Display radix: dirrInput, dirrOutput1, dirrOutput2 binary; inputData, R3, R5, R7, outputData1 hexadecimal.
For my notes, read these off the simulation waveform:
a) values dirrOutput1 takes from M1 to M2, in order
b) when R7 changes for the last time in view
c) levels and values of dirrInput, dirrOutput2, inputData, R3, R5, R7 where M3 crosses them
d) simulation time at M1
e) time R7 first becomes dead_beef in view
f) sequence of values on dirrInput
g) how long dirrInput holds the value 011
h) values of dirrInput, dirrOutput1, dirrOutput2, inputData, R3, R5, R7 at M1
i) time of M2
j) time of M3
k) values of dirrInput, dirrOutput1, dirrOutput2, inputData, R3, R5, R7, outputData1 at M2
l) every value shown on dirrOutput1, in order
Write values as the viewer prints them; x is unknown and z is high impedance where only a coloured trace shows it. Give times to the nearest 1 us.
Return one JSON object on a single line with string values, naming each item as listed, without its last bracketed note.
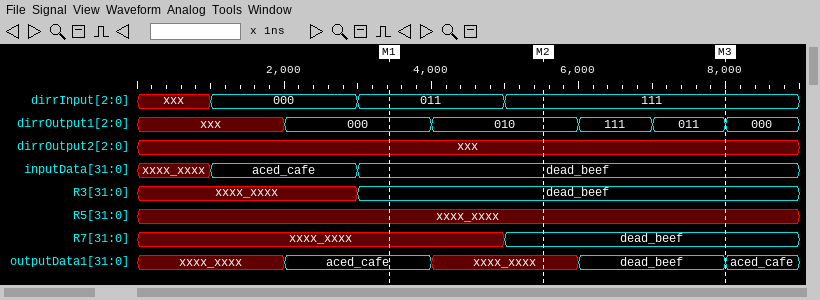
{"values dirrOutput1 takes from M1 to M2, in order": "000, 010", "when R7 changes for the last time in view": "5 us", "levels and values of dirrInput, dirrOutput2, inputData, R3, R5, R7 where M3 crosses them": "dirrInput=111, dirrOutput2=xxx, inputData=dead_beef, R3=dead_beef, R5=xxxx_xxxx, R7=dead_beef", "simulation time at M1": "3 us", "time R7 first becomes dead_beef in view": "5 us", "sequence of values on dirrInput": "xxx, 000, 011, 111", "how long dirrInput holds the value 011": "2 us", "values of dirrInput, dirrOutput1, dirrOutput2, inputData, R3, R5, R7 at M1": "dirrInput=011, dirrOutput1=000, dirrOutput2=xxx, inputData=dead_beef, R3=dead_beef, R5=xxxx_xxxx, R7=xxxx_xxxx", "time of M2": "6 us", "time of M3": "8 us", "values of dirrInput, dirrOutput1, dirrOutput2, inputData, R3, R5, R7, outputData1 at M2": "dirrInput=111, dirrOutput1=010, dirrOutput2=xxx, inputData=dead_beef, R3=dead_beef, R5=xxxx_xxxx, R7=dead_beef, outputData1=xxxx_xxxx", "every value shown on dirrOutput1, in order": "xxx, 000, 010, 111, 011, 000"}
